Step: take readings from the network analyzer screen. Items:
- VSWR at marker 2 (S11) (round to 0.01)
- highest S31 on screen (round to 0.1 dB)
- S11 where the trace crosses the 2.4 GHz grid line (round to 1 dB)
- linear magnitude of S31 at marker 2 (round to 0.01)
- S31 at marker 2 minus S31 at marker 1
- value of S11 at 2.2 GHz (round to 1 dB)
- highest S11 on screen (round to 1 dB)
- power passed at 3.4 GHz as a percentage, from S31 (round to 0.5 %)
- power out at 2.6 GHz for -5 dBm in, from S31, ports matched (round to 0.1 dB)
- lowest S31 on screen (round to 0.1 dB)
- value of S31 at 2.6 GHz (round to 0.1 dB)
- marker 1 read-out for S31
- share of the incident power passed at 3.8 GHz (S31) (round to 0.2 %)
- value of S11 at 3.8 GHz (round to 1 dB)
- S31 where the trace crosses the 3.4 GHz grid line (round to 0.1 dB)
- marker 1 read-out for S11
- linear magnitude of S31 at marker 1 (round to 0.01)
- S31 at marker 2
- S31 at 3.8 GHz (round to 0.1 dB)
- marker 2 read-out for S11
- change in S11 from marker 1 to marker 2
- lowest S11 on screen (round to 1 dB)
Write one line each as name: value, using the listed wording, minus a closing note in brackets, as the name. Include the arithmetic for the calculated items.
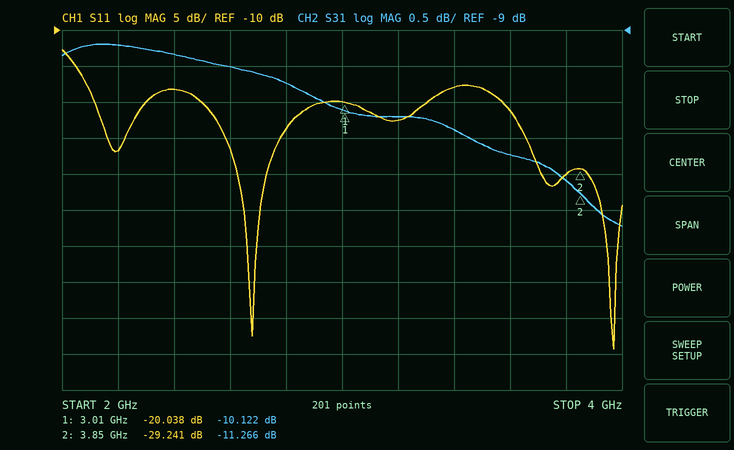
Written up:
VSWR at marker 2 (S11): (1 + 0.0345)/(1 − 0.0345) ≈ 1.07
highest S31 on screen: -9.2 dB
S11 where the trace crosses the 2.4 GHz grid line: -18 dB
linear magnitude of S31 at marker 2: 10^(-11.266/20) ≈ 0.27
S31 at marker 2 minus S31 at marker 1: -11.266 − (-10.122) = -1.144 dB
value of S11 at 2.2 GHz: -27 dB
highest S11 on screen: -13 dB
power passed at 3.4 GHz as a percentage, from S31: 10^(-10.4/10) ≈ 9.12 %, so 9.0 % to the nearest 0.5 %
power out at 2.6 GHz for -5 dBm in, from S31, ports matched: -5 dBm + (-9.5 dB) = -14.5 dBm
lowest S31 on screen: -11.7 dB
value of S31 at 2.6 GHz: -9.5 dB
marker 1 read-out for S31: -10.122 dB
share of the incident power passed at 3.8 GHz (S31): 10^(-11.1/10) ≈ 7.8 %
value of S11 at 3.8 GHz: -30 dB
S31 where the trace crosses the 3.4 GHz grid line: -10.4 dB
marker 1 read-out for S11: -20.038 dB
linear magnitude of S31 at marker 1: 10^(-10.122/20) ≈ 0.31
S31 at marker 2: -11.266 dB
S31 at 3.8 GHz: -11.1 dB
marker 2 read-out for S11: -29.241 dB
change in S11 from marker 1 to marker 2: -29.241 − (-20.038) = -9.203 dB
lowest S11 on screen: -54 dB
